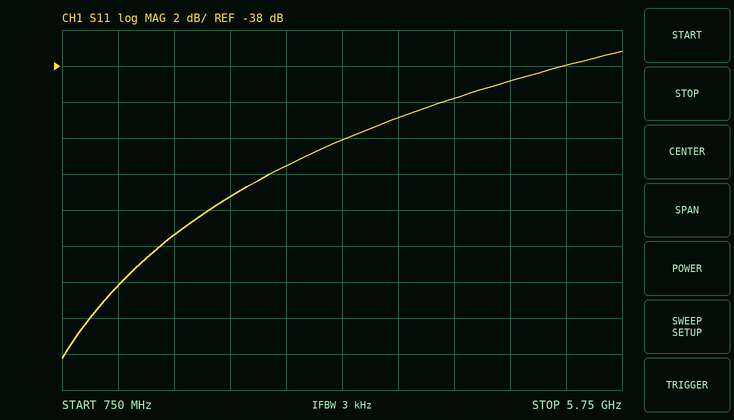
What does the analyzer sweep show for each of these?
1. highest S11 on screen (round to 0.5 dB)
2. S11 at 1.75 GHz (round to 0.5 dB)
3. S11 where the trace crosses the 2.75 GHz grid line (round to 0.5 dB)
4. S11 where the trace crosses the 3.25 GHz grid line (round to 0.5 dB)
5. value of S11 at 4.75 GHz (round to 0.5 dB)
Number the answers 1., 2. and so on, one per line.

1. -37.0 dB
2. -47.5 dB
3. -43.5 dB
4. -42.0 dB
5. -39.0 dB
